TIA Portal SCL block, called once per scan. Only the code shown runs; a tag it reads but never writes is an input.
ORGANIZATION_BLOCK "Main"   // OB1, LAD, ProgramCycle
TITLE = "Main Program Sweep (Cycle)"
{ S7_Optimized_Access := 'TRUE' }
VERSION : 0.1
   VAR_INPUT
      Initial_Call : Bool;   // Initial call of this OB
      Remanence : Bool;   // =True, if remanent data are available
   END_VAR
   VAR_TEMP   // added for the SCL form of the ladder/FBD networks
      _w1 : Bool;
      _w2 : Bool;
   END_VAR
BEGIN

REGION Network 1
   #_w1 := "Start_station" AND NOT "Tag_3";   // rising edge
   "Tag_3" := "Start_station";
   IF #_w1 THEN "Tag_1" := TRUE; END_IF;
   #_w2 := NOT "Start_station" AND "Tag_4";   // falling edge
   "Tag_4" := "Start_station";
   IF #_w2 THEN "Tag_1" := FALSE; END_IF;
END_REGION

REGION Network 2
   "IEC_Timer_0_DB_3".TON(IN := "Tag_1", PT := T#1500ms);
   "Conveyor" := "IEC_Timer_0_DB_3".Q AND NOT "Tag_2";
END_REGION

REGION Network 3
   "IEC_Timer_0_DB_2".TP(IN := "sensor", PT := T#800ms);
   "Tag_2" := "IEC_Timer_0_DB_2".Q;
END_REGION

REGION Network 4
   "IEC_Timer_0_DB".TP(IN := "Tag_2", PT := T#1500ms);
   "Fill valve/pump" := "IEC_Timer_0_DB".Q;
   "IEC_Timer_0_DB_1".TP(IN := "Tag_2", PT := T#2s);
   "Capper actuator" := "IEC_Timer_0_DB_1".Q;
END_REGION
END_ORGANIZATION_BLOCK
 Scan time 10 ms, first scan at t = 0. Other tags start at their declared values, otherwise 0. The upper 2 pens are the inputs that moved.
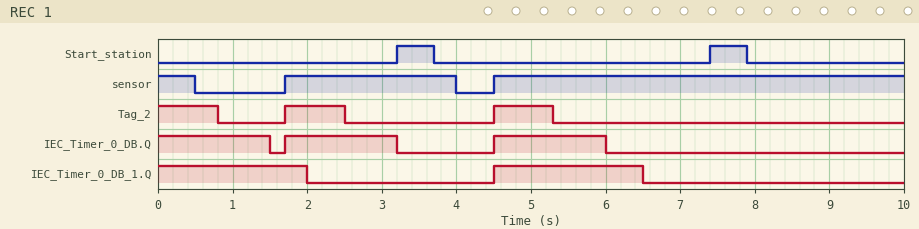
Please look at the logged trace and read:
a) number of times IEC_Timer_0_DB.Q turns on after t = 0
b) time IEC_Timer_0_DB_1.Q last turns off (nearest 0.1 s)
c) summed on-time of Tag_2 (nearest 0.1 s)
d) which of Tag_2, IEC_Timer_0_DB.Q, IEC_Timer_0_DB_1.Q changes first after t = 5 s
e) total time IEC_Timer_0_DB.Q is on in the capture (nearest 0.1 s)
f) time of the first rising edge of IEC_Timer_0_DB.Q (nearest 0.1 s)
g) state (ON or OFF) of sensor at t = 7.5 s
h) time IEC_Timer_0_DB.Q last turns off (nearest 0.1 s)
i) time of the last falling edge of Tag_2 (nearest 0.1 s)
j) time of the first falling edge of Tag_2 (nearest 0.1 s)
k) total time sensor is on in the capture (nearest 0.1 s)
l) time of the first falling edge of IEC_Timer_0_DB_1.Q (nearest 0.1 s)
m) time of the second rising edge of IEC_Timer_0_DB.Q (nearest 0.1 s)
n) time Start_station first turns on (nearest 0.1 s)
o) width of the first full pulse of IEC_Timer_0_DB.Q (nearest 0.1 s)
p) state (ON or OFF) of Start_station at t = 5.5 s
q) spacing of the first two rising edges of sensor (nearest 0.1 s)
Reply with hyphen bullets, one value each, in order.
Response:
- 2
- 6.5 s
- 2.4 s
- Tag_2
- 4.5 s
- 1.7 s
- ON
- 6.0 s
- 5.3 s
- 0.8 s
- 8.3 s
- 2.0 s
- 4.5 s
- 3.2 s
- 1.5 s
- OFF
- 2.8 s
